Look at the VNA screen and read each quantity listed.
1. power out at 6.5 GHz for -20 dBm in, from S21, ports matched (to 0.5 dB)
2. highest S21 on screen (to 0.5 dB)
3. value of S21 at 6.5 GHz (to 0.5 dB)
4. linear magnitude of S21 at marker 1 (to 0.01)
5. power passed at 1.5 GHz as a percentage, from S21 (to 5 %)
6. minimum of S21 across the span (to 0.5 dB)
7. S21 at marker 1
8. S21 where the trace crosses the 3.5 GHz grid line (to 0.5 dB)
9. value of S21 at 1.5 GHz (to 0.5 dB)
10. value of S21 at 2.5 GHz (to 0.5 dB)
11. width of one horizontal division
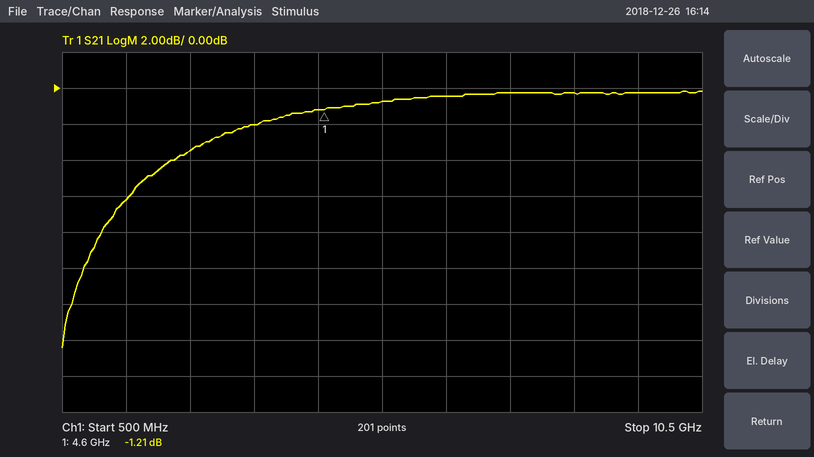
-20.5 dBm
0.0 dB
-0.5 dB
0.87
25 %
-14.5 dB
-1.21 dB
-2.0 dB
-6.0 dB
-3.5 dB
1 GHz
